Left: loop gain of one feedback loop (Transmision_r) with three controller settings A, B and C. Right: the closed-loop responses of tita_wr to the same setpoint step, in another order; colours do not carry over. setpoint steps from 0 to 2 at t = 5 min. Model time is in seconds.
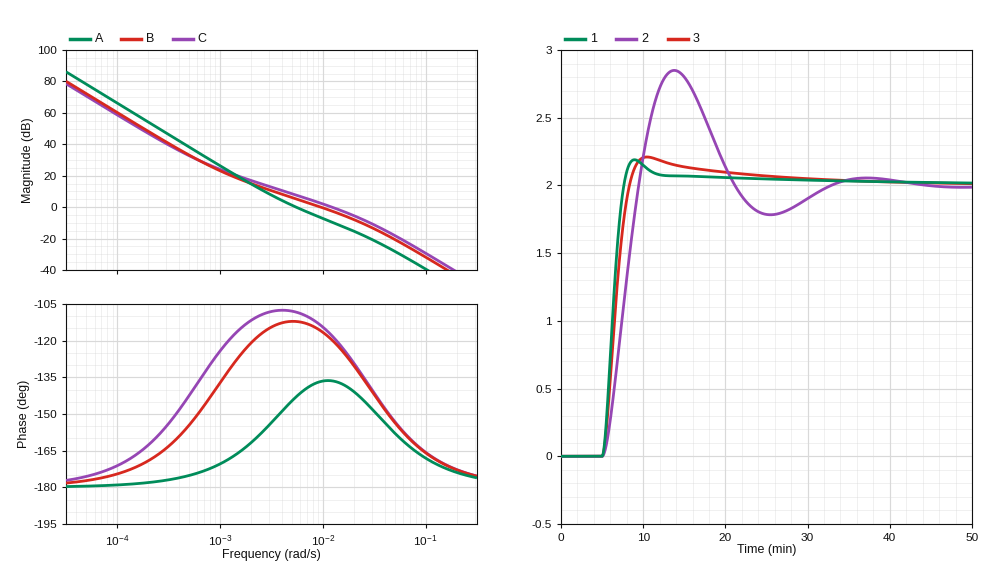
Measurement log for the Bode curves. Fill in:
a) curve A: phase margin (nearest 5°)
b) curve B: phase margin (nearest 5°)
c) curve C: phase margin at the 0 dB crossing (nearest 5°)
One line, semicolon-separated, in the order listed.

35°; 65°; 60°
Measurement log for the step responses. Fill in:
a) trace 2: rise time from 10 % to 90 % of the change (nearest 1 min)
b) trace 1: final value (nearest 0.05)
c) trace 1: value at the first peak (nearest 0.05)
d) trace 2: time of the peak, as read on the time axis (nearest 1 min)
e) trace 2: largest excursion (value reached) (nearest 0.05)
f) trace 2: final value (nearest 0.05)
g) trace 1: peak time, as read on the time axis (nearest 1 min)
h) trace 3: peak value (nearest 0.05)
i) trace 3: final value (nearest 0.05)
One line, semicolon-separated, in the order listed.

3 min; 2.00; 2.20; 14 min; 2.85; 2.00; 9 min; 2.20; 2.00
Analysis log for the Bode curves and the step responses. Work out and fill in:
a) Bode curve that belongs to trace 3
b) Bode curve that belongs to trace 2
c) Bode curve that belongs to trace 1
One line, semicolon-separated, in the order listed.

B; A; C
